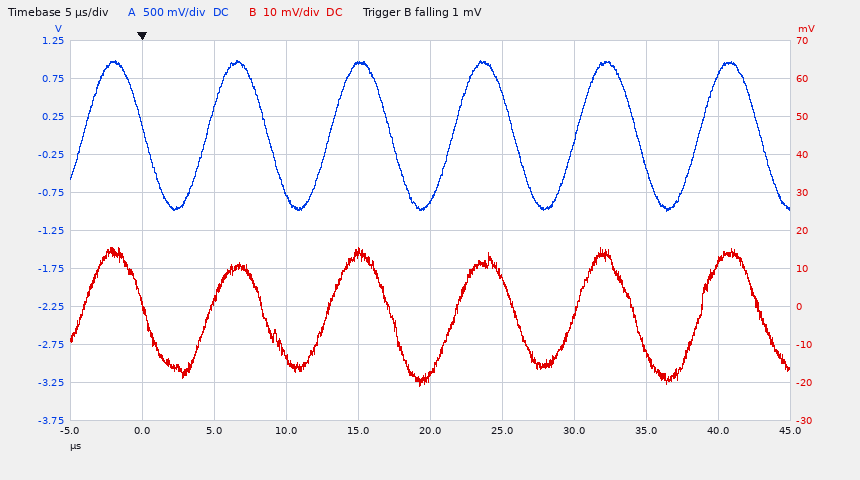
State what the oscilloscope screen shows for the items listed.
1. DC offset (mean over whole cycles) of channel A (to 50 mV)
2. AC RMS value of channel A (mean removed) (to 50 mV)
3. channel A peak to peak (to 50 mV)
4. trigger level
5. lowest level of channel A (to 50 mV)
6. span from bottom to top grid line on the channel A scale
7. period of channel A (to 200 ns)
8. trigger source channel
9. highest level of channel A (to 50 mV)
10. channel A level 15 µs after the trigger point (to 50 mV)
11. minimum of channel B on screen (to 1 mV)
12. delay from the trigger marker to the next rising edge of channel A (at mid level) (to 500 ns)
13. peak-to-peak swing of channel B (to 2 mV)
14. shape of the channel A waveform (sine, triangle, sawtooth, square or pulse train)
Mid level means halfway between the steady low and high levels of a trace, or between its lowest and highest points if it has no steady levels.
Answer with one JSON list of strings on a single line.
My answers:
["0 mV", "700 mV", "2.00 V", "1 mV", "-1.00 V", "5 V", "8.6 µs", "channel B", "1.00 V", "950 mV", "-21 mV", "4.5 µs", "36 mV", "sine"]
